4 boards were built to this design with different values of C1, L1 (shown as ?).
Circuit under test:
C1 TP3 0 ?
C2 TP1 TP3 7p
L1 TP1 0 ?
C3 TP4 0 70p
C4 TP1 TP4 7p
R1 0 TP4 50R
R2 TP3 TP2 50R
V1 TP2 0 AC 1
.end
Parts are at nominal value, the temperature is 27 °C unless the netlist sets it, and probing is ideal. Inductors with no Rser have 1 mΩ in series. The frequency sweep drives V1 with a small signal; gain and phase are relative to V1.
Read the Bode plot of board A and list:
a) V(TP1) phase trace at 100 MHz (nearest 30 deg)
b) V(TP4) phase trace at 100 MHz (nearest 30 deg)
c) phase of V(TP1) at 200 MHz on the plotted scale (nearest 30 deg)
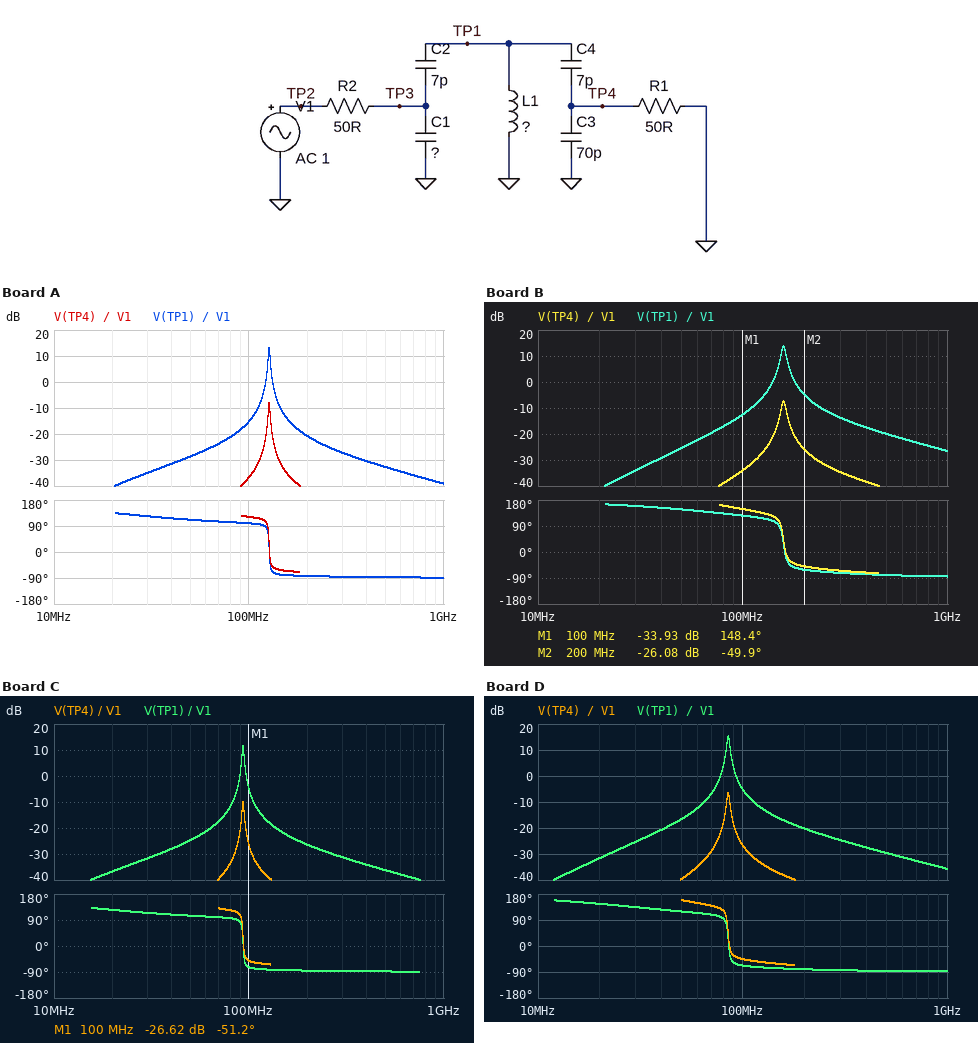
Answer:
90 deg
120 deg
-90 deg
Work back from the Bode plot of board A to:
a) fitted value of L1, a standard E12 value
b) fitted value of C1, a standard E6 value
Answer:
120 nH
150 pF
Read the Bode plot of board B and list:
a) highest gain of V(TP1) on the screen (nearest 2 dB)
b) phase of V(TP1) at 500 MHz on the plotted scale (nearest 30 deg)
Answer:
14 dB
-90 deg
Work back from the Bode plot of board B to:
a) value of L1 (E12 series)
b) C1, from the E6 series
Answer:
82 nH
33 pF
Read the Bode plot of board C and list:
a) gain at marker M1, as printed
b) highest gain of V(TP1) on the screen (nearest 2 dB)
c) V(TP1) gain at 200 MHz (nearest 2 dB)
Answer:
-26.62 dB
12 dB
-26 dB
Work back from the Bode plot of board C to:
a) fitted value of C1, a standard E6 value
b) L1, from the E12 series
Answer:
220 pF
220 nH
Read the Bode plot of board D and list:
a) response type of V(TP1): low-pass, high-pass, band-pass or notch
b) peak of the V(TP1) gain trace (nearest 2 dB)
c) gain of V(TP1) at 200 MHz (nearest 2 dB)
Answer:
band-pass
16 dB
-20 dB
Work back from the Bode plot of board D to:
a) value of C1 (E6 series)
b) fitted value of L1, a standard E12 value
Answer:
100 pF
270 nH
